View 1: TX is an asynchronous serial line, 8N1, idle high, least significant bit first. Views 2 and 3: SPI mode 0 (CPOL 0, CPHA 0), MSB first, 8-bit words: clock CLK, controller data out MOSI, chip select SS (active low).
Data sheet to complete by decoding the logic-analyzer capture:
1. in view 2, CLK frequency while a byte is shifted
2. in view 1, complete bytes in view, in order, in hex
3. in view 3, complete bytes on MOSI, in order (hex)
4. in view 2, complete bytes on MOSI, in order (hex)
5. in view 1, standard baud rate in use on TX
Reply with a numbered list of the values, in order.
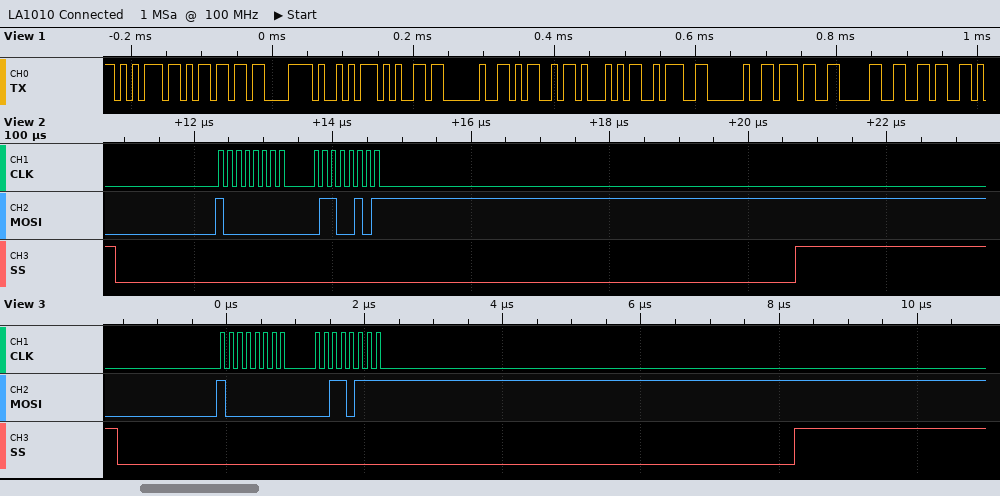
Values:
1. 8 MHz
2. 0x75 0x6D 0xC3 0xA9 0x65 0x20 0x4D 0x51 0x3A 0x20 0x37 0x30 0x36
3. 0x80 0x37
4. 80 65
5. 115200 baud
